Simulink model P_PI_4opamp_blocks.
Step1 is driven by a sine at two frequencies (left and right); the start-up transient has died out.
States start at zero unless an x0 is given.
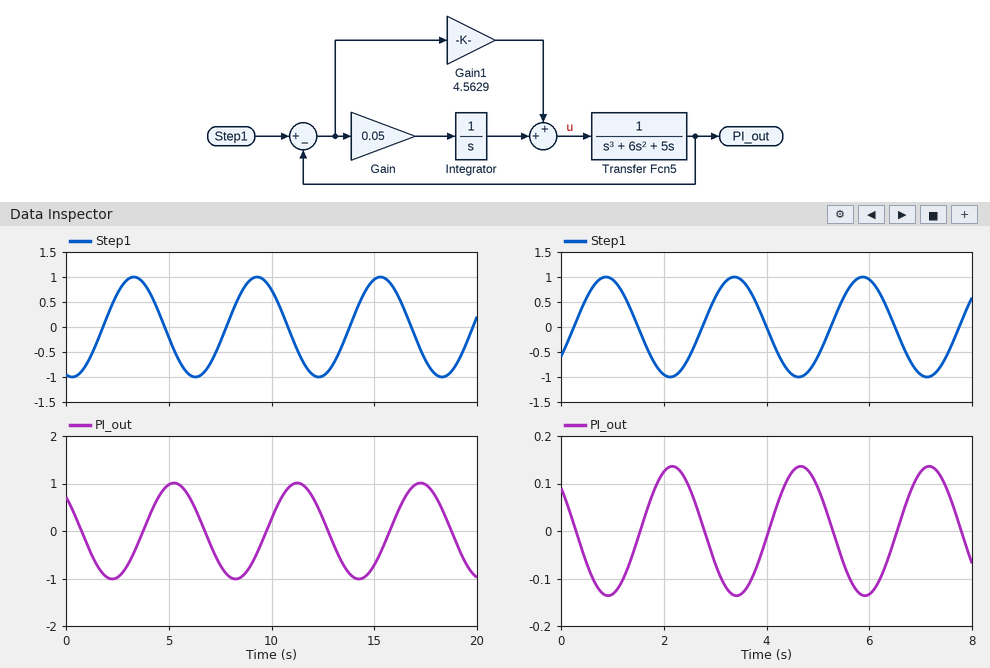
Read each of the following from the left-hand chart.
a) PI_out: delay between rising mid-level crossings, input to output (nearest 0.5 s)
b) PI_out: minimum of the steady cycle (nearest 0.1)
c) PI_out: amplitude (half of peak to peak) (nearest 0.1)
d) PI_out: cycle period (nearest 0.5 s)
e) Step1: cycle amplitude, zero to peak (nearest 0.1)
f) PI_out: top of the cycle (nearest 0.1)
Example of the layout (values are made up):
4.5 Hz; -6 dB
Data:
2.0 s; -1.0; 1.0; 6.0 s; 1.0; 1.0
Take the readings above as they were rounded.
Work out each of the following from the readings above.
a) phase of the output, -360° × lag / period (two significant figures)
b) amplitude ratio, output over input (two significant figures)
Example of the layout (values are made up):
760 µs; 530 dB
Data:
-120°; 1.0
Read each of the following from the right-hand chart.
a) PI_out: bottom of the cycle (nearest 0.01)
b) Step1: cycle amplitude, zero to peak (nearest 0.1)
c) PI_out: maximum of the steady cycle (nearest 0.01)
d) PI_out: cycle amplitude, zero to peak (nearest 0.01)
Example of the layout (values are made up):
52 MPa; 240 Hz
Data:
-0.14; 1.0; 0.14; 0.14
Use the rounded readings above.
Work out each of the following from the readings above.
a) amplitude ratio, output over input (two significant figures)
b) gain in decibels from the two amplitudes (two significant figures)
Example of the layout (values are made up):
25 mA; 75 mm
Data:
0.14; -17 dB
